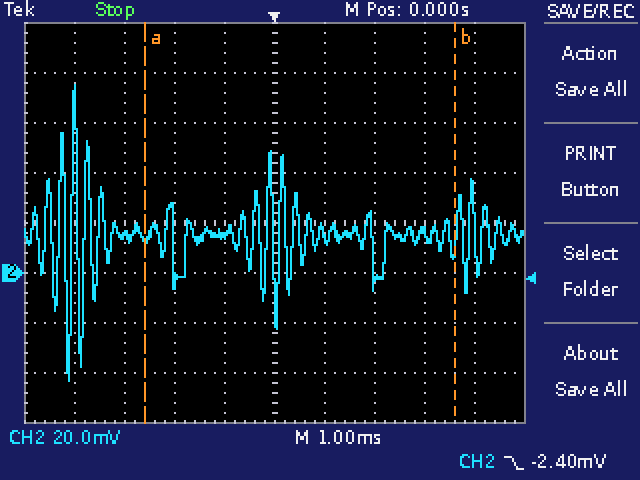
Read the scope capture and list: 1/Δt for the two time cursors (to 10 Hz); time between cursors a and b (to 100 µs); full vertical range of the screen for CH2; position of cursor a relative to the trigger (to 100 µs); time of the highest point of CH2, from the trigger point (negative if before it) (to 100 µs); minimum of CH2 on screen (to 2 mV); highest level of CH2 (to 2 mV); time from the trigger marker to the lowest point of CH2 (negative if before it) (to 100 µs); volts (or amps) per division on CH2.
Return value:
160 Hz
6.2 ms
160 mV
-2.6 ms
-4.0 ms
-44 mV
76 mV
-4.1 ms
20 mV
